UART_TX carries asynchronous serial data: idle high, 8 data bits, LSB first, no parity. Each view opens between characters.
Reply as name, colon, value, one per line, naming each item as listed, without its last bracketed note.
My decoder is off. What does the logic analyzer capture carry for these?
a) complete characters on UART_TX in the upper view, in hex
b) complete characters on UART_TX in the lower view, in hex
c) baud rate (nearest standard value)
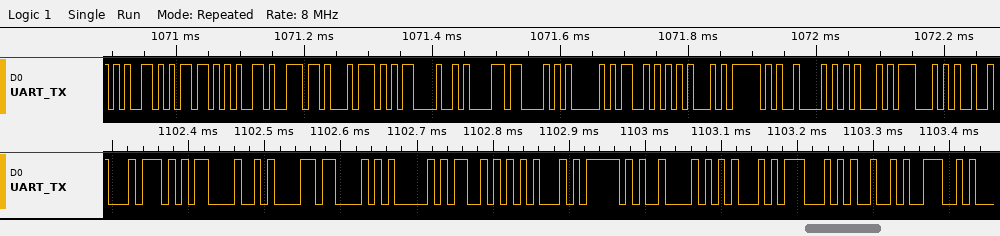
complete characters on UART_TX in the upper view, in hex: 65, 6D, 65, 6E, 74, 0D, 0A, 43, 41, 53, 45, 5F, 42, 45, 47
complete characters on UART_TX in the lower view, in hex: 74, 0D, 0A, 43, 41, 53, 45, 5F, 42, 45, 47, 49, 4E
baud rate: 115200 baud
